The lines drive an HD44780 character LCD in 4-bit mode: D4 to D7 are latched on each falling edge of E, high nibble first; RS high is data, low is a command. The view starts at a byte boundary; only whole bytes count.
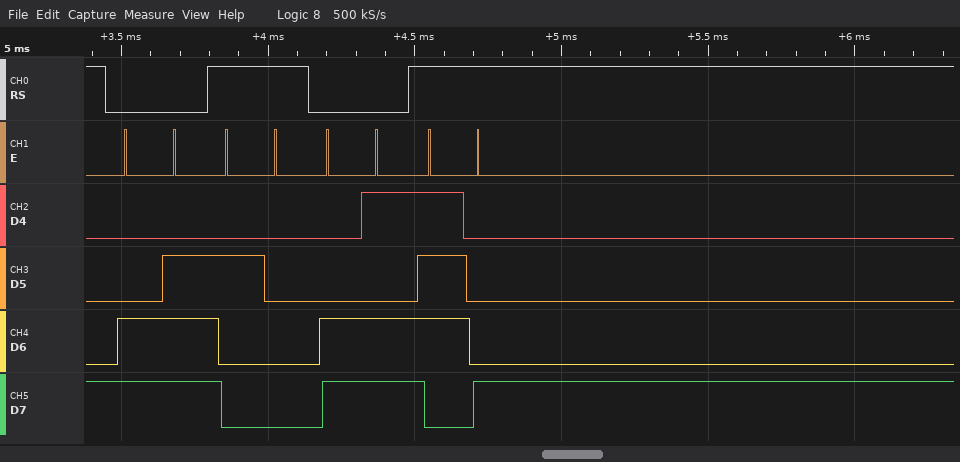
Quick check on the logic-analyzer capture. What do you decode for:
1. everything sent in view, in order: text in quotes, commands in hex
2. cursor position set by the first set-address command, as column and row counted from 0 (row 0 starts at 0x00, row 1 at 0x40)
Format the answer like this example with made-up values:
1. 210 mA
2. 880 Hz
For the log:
1. 0xCE " " 0xCD "x"
2. column 14, row 1
